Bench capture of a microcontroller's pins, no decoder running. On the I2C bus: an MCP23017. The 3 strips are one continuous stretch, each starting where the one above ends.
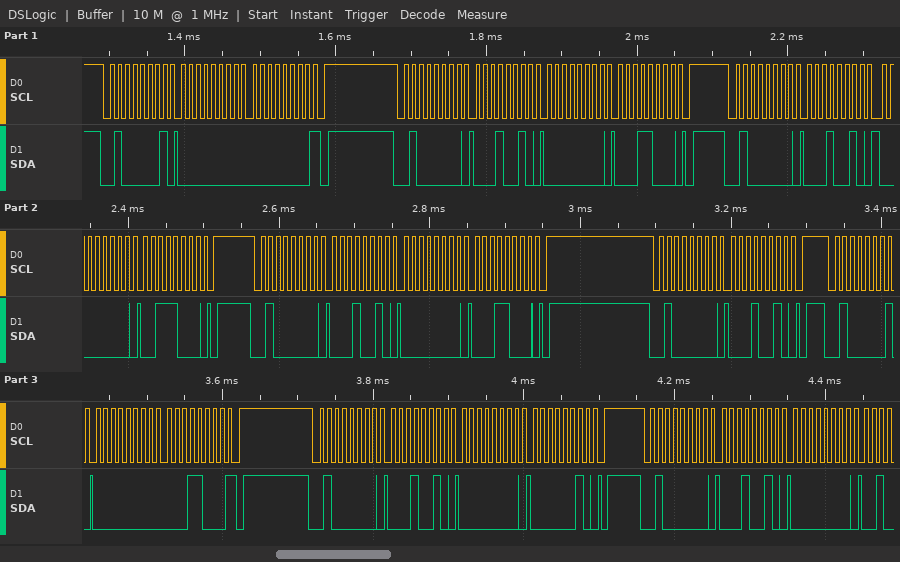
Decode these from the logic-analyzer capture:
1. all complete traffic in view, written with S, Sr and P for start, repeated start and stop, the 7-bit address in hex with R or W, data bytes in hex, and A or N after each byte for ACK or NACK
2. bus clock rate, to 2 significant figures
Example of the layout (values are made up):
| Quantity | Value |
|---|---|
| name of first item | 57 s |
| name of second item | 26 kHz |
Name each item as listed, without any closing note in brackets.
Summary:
| Quantity | Value |
|---|---|
| all complete traffic in view, written with S, Sr and P for start, repeated start and stop, the 7-bit address in hex with R or W, data bytes in hex, and A or N after each byte for ACK or NACK | S 20R A 00 A 00 N P S 20W A 12 A 00 A 18 A P S 20W A 12 A 00 A 38 A P S 20W A 12 A 00 A 18 A P S 20W A 12 A P S 20R A 00 A 18 N P S 20W A 12 A 00 A 02 A P S 20W A 12 A 00 A |
| bus clock rate, to 2 significant figures | 100 kHz |
